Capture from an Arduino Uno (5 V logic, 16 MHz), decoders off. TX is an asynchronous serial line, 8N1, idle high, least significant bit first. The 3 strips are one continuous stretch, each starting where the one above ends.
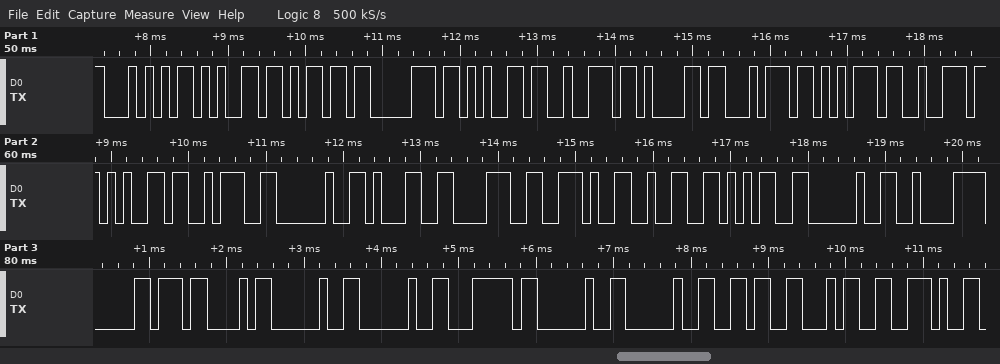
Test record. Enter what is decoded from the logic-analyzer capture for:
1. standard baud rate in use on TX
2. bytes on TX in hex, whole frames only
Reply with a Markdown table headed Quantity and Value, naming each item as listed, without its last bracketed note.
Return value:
| Quantity | Value |
|---|---|
| standard baud rate in use on TX | 9600 baud |
| bytes on TX in hex, whole frames only | 0x54 0x65 0x6D 0x70 0x65 0x72 0x61 0x74 0x75 0x72 0x65 0x3A 0x20 0x31 0x38 0x2E 0x32 0x35 0x20 0xC2 0xB0 0x43 0x20 0x20 0x7C 0x20 0x20 0x36 0x34 0x2E |
